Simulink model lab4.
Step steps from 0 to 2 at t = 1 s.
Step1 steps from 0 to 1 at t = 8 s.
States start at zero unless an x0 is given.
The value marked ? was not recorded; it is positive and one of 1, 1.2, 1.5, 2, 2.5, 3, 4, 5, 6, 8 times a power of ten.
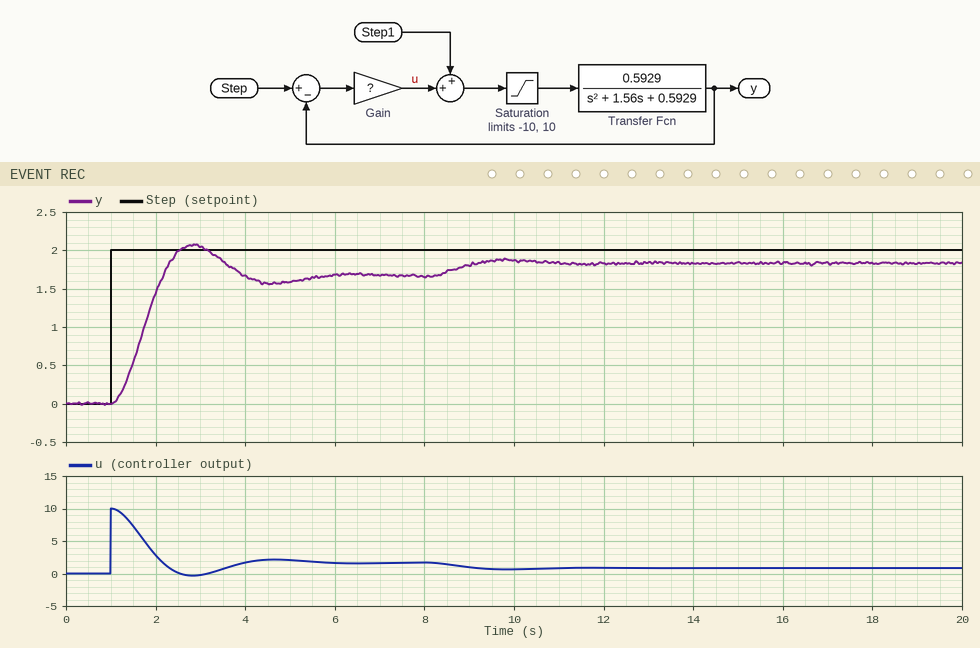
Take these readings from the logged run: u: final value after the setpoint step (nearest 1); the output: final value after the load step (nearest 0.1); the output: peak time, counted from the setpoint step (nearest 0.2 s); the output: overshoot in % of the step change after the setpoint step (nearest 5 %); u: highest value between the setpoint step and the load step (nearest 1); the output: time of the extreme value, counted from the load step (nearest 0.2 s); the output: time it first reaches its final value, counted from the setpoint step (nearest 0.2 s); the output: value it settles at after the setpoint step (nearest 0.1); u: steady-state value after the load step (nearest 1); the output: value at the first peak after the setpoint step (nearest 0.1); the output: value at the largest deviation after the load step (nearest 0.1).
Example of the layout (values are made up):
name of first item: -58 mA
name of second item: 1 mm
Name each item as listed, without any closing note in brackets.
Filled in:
u: final value after the setpoint step: 2
the output: final value after the load step: 1.8
the output: peak time, counted from the setpoint step: 1.8 s
the output: overshoot in % of the step change after the setpoint step: 25 %
u: highest value between the setpoint step and the load step: 10
the output: time of the extreme value, counted from the load step: 1.8 s
the output: time it first reaches its final value, counted from the setpoint step: 1.2 s
the output: value it settles at after the setpoint step: 1.7
u: steady-state value after the load step: 1
the output: value at the first peak after the setpoint step: 2.1
the output: value at the largest deviation after the load step: 1.9
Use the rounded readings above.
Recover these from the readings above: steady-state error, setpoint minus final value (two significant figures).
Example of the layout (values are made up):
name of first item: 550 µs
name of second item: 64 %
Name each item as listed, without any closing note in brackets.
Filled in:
steady-state error, setpoint minus final value: 0.30
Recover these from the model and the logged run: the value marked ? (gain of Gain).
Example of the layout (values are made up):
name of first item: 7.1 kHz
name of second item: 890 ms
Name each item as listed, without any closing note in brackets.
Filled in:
the value marked ?: 5
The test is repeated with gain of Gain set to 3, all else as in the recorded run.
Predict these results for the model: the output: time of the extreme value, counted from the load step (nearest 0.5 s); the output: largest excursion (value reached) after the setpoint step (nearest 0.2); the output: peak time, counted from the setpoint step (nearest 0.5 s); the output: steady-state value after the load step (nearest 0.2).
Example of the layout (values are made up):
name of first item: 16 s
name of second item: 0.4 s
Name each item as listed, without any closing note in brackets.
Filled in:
the output: time of the extreme value, counted from the load step: 2.5 s
the output: largest excursion (value reached) after the setpoint step: 1.8
the output: peak time, counted from the setpoint step: 2.5 s
the output: steady-state value after the load step: 1.8
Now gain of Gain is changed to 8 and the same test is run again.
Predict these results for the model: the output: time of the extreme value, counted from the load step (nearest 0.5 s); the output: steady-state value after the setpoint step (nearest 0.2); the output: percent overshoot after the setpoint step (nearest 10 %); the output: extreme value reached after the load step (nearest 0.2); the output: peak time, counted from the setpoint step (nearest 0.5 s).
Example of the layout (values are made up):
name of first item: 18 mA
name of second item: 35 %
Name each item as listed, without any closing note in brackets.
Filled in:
the output: time of the extreme value, counted from the load step: 1.5 s
the output: steady-state value after the setpoint step: 1.8
the output: percent overshoot after the setpoint step: 30 %
the output: extreme value reached after the load step: 2.0
the output: peak time, counted from the setpoint step: 1.5 s
